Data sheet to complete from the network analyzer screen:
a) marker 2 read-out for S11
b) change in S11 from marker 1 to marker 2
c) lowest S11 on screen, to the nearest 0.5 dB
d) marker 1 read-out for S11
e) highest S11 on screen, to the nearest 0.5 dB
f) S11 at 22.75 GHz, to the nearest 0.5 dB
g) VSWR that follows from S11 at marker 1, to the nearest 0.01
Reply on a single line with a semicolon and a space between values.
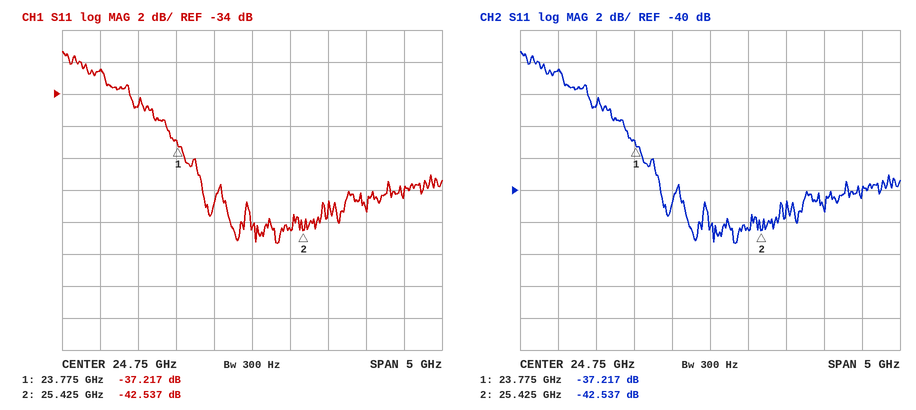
-42.537 dB; -5.320 dB; -43.5 dB; -37.217 dB; -31.5 dB; -32.5 dB; 1.03
